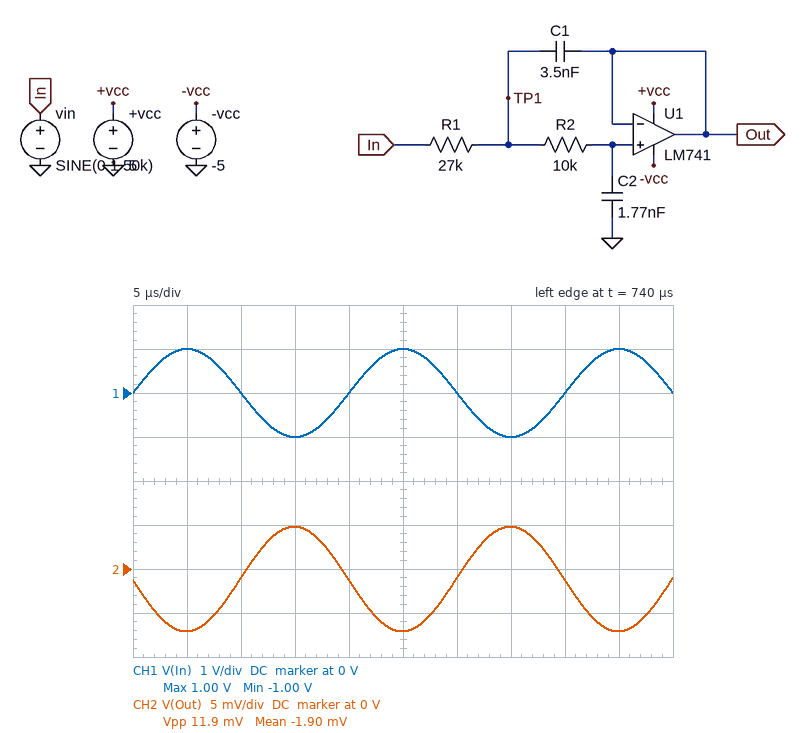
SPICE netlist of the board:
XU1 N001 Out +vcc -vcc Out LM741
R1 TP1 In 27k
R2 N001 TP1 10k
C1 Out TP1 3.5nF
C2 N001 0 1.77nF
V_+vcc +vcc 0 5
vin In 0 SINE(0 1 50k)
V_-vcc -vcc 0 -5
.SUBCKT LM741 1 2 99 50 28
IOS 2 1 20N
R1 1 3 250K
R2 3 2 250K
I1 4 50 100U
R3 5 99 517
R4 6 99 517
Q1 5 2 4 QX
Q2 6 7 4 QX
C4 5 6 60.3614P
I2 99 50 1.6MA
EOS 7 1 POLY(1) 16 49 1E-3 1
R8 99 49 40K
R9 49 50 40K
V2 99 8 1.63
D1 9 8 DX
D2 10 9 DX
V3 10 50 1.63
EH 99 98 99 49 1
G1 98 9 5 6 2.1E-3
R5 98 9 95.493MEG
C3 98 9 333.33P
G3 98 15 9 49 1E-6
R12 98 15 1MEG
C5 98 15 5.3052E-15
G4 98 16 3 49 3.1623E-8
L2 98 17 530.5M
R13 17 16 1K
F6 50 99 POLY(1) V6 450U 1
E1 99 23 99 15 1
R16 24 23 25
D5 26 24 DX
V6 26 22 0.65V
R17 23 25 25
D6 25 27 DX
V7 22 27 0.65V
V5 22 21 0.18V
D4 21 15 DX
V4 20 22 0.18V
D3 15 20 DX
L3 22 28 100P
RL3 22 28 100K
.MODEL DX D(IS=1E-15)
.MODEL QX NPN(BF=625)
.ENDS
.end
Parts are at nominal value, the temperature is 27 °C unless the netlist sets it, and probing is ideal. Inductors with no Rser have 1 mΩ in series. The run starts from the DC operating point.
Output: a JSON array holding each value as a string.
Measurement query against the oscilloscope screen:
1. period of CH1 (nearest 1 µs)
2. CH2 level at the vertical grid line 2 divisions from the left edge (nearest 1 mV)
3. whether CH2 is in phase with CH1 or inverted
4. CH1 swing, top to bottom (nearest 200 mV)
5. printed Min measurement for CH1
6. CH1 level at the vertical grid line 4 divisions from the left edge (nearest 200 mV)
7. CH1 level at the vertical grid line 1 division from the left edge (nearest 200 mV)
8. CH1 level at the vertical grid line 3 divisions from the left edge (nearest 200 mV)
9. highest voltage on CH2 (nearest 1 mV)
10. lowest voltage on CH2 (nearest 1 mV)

["20 µs", "-1 mV", "inverted", "2.0 V", "-1.00 V", "0 V", "1.0 V", "-1.0 V", "5 mV", "-7 mV"]
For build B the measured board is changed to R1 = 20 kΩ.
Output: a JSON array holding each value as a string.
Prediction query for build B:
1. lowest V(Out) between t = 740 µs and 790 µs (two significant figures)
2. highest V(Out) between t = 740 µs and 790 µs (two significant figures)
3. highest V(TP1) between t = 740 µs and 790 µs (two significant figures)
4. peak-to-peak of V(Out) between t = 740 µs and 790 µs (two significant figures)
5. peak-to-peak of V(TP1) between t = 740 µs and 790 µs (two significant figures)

["-8.8 mV", "7.3 mV", "44 mV", "16 mV", "91 mV"]
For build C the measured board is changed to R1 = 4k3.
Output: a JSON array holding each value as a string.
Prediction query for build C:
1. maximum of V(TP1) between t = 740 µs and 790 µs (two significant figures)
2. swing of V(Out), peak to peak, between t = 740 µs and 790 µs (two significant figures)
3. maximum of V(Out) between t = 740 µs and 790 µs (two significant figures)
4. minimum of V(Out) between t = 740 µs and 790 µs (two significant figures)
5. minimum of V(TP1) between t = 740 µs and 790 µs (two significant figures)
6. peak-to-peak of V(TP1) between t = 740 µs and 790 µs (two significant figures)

["210 mV", "74 mV", "37 mV", "-37 mV", "-210 mV", "420 mV"]
